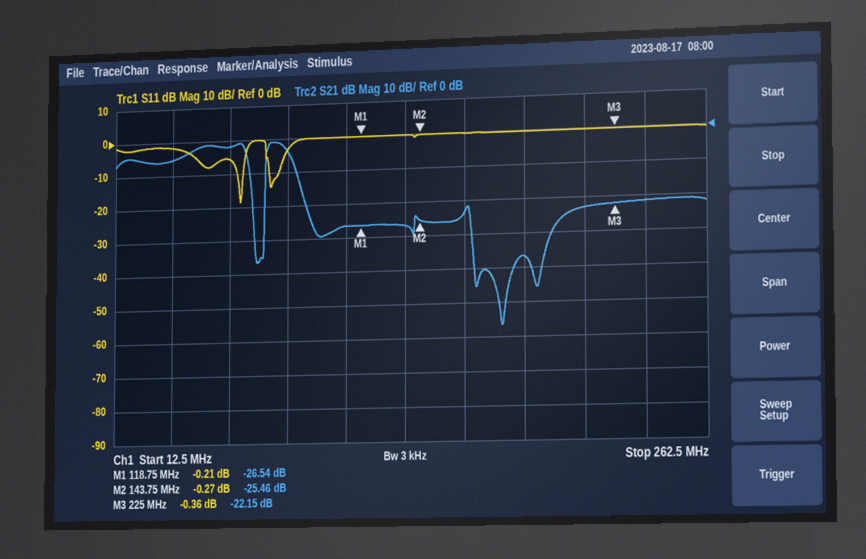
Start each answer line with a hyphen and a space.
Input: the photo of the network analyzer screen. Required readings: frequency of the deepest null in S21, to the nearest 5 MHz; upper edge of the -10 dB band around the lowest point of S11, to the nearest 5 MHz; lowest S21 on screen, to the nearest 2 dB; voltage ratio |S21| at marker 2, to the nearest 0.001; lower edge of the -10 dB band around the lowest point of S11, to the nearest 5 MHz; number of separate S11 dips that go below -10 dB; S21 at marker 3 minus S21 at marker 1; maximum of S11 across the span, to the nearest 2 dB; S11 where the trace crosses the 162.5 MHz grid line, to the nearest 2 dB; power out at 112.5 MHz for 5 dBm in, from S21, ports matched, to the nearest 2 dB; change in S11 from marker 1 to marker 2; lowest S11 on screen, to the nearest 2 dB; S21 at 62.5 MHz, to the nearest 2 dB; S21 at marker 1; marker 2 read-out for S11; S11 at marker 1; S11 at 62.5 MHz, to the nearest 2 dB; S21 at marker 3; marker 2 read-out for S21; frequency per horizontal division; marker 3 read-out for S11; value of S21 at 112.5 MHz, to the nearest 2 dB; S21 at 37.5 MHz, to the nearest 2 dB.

- 180 MHz
- 70 MHz
- -56 dB
- 0.053
- 65 MHz
- 2
- 4.39 dB
- 0 dB
- 0 dB
- -22 dBm
- -0.06 dB
- -18 dB
- -2 dB
- -26.54 dB
- -0.27 dB
- -0.21 dB
- -6 dB
- -22.15 dB
- -25.46 dB
- 25 MHz
- -0.36 dB
- -26 dB
- -6 dB
